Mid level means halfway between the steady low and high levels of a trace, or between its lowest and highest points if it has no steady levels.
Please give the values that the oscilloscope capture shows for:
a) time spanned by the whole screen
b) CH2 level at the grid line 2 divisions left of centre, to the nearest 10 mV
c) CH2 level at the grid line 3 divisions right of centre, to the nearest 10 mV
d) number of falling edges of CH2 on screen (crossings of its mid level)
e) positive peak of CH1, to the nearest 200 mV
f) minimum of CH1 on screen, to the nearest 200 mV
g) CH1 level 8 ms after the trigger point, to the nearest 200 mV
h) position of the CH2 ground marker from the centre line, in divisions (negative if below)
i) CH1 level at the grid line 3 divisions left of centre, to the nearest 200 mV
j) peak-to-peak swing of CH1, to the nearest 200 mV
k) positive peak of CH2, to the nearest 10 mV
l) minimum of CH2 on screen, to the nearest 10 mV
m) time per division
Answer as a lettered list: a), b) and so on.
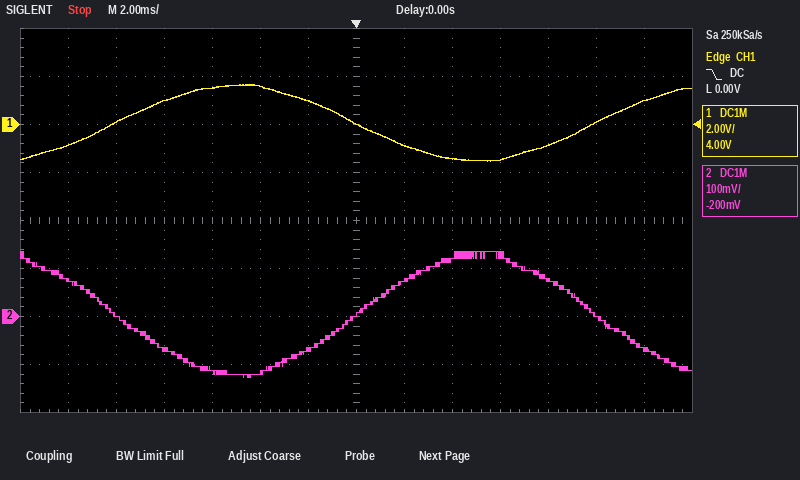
a) 28 ms
b) -120 mV
c) 130 mV
d) 2
e) 1.6 V
f) -1.6 V
g) -800 mV
h) -2.0 div
i) 1.6 V
j) 3.2 V
k) 140 mV
l) -130 mV
m) 2 ms
